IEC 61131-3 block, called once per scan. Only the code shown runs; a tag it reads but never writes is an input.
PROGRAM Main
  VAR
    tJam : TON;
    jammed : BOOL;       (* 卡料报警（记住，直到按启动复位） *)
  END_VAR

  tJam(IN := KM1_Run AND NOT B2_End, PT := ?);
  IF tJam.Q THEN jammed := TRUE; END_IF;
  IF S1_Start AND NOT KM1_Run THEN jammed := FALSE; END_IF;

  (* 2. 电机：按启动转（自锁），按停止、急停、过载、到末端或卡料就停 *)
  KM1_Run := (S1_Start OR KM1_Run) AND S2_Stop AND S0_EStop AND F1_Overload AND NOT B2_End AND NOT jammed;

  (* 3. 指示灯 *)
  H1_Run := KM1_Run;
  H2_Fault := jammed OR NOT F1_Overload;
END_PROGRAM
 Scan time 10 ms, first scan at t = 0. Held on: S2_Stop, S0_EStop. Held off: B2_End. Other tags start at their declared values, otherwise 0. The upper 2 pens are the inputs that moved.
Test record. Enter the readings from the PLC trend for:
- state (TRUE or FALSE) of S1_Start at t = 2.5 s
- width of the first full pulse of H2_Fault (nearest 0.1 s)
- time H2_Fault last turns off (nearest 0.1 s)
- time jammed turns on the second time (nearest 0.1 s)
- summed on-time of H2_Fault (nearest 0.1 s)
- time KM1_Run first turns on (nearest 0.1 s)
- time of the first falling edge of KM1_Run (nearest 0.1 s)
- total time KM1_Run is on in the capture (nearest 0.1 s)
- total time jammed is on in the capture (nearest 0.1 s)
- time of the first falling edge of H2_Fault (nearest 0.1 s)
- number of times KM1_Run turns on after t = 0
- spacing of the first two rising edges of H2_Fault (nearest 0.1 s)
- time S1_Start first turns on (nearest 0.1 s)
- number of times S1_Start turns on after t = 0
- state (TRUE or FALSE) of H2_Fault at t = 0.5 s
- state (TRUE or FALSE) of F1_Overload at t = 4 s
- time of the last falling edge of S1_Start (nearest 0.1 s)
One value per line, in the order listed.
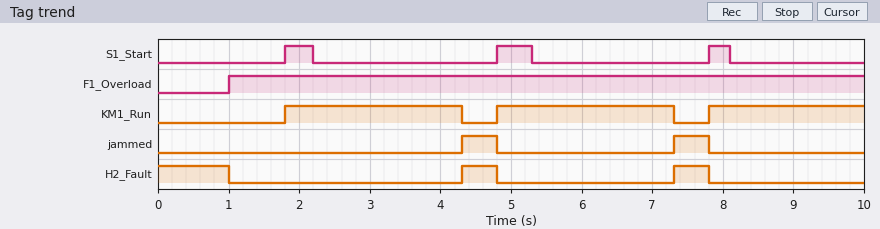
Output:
FALSE
0.5 s
7.8 s
7.3 s
2.0 s
1.8 s
4.3 s
7.2 s
1.0 s
1.0 s
3
3.0 s
1.8 s
3
TRUE
TRUE
8.1 s
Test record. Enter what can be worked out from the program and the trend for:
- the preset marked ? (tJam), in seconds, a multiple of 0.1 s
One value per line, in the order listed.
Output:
2.5 s
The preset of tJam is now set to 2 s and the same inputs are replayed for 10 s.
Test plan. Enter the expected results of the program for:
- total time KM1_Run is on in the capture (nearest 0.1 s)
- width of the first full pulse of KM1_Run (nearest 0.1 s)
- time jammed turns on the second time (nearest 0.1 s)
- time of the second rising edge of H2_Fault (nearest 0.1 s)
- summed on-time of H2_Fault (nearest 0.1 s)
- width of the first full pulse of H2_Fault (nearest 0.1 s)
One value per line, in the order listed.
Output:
6.0 s
2.0 s
6.8 s
6.8 s
3.2 s
1.0 s
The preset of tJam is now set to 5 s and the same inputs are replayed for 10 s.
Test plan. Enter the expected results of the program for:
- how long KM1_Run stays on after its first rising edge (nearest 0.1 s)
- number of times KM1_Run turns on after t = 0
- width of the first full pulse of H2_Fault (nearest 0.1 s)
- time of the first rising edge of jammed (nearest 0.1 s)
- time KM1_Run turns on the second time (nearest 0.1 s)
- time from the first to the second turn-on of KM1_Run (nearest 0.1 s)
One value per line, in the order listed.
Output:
5.0 s
2
1.0 s
6.8 s
7.8 s
6.0 s
